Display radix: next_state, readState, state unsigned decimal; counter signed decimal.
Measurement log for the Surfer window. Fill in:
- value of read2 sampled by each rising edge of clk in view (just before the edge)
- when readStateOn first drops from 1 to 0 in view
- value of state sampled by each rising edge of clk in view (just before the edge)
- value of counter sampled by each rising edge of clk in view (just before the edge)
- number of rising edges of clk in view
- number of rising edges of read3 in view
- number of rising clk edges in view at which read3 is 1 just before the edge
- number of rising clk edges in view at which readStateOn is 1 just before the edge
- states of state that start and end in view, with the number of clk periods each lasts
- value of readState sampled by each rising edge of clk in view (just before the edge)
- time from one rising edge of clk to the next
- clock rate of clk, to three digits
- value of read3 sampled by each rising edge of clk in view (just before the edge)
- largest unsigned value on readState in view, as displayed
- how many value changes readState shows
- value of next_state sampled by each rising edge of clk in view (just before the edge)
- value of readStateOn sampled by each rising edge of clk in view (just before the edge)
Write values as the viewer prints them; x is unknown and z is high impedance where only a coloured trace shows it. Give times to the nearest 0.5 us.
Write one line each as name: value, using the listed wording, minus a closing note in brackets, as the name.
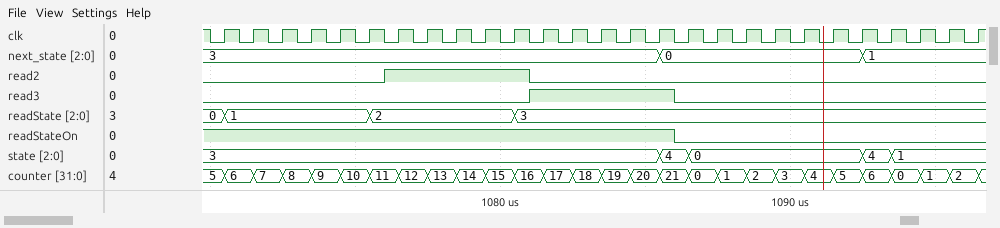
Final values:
value of read2 sampled by each rising edge of clk in view: 0 0 0 0 0 0 1 1 1 1 1 0 0 0 0 0 0 0 0 0 0 0 0 0 0 0 0
when readStateOn first drops from 1 to 0 in view: 1086 us
value of state sampled by each rising edge of clk in view: 3, 3, 3, 3, 3, 3, 3, 3, 3, 3, 3, 3, 3, 3, 3, 3, 4, 0, 0, 0, 0, 0, 0, 4, 1, 1, 1
value of counter sampled by each rising edge of clk in view: 5, 6, 7, 8, 9, 10, 11, 12, 13, 14, 15, 16, 17, 18, 19, 20, 21, 0, 1, 2, 3, 4, 5, 6, 0, 1, 2
number of rising edges of clk in view: 27
number of rising edges of read3 in view: 1
number of rising clk edges in view at which read3 is 1 just before the edge: 5
number of rising clk edges in view at which readStateOn is 1 just before the edge: 16
states of state that start and end in view, with the number of clk periods each lasts: 4: 1, 0: 6, 4: 1
value of readState sampled by each rising edge of clk in view: 0, 1, 1, 1, 1, 1, 2, 2, 2, 2, 2, 3, 3, 3, 3, 3, 3, 3, 3, 3, 3, 3, 3, 3, 3, 3, 3
time from one rising edge of clk to the next: 1 us
clock rate of clk, to three digits: 1.00 MHz
value of read3 sampled by each rising edge of clk in view: 0 0 0 0 0 0 0 0 0 0 0 1 1 1 1 1 0 0 0 0 0 0 0 0 0 0 0
largest unsigned value on readState in view, as displayed: 3
how many value changes readState shows: 3
value of next_state sampled by each rising edge of clk in view: 3, 3, 3, 3, 3, 3, 3, 3, 3, 3, 3, 3, 3, 3, 3, 3, 0, 0, 0, 0, 0, 0, 0, 1, 1, 1, 1
value of readStateOn sampled by each rising edge of clk in view: 1 1 1 1 1 1 1 1 1 1 1 1 1 1 1 1 0 0 0 0 0 0 0 0 0 0 0
